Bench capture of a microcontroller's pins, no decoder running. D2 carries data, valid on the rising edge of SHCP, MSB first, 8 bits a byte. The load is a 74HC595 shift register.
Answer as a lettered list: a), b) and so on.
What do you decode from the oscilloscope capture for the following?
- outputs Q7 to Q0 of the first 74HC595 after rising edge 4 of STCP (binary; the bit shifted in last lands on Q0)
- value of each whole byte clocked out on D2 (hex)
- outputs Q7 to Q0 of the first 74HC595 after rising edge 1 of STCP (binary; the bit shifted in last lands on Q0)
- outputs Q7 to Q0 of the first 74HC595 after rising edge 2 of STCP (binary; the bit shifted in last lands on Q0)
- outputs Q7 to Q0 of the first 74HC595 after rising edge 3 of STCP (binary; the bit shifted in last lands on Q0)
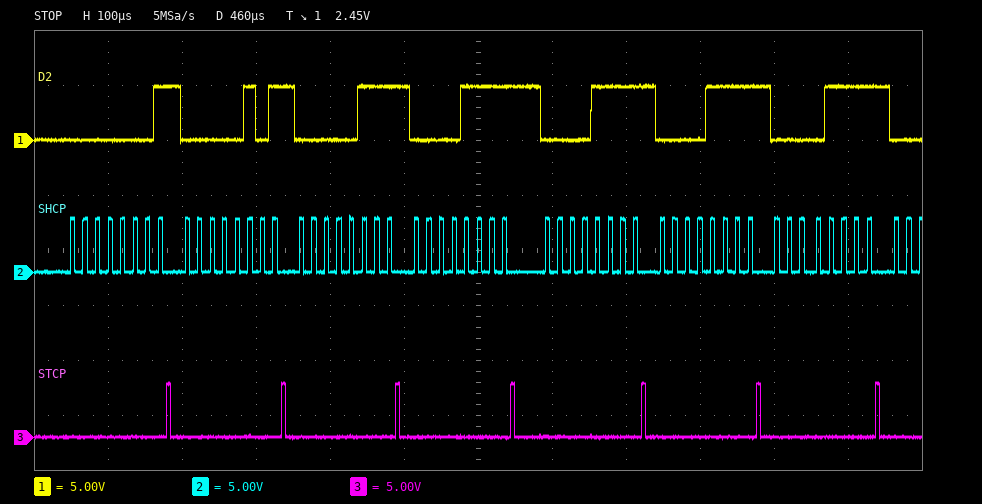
a) 00001111
b) 01 05 07 0F 0F 0F 0F
c) 00000001
d) 00000101
e) 00000111
